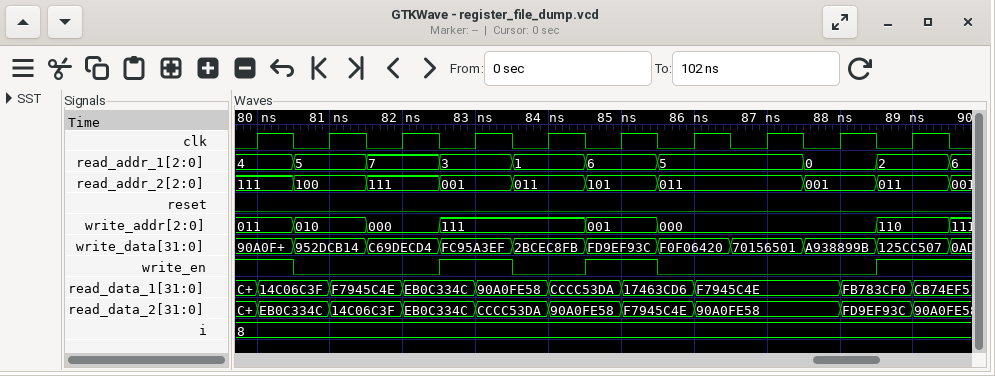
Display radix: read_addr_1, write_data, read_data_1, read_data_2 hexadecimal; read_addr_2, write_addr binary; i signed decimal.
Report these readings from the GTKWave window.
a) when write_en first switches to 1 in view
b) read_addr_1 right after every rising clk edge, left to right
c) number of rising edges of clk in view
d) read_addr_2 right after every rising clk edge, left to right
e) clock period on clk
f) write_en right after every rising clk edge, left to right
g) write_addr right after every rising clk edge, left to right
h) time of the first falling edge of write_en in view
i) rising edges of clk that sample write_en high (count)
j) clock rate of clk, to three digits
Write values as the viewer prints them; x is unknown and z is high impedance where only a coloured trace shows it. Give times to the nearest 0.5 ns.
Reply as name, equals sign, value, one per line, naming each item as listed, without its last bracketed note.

when write_en first switches to 1 in view = 82.5 ns
read_addr_1 right after every rising clk edge, left to right = 4, 5, 7, 3, 1, 6, 5, 5, 0, 2
number of rising edges of clk in view = 10
read_addr_2 right after every rising clk edge, left to right = 111, 100, 111, 001, 011, 101, 011, 011, 001, 011
clock period on clk = 1 ns
write_en right after every rising clk edge, left to right = 1 0 0 1 0 1 0 0 0 1
write_addr right after every rising clk edge, left to right = 011, 010, 000, 111, 111, 001, 000, 000, 000, 110
time of the first falling edge of write_en in view = 80.5 ns
rising edges of clk that sample write_en high = 4
clock rate of clk, to three digits = 1.00 GHz
